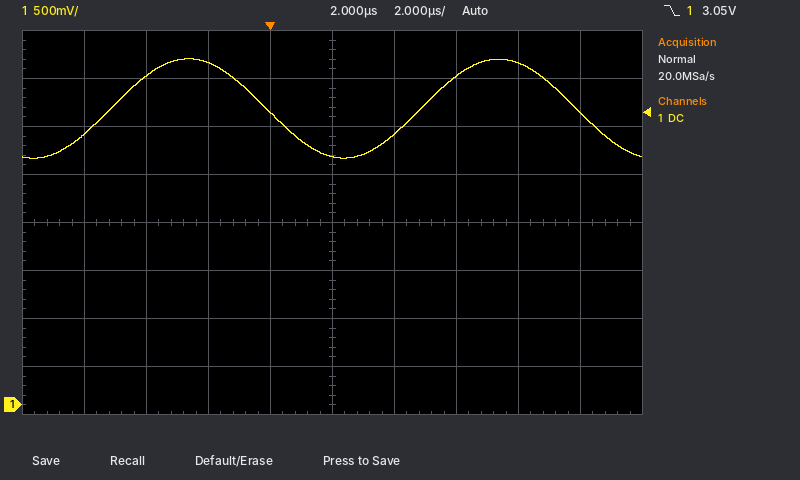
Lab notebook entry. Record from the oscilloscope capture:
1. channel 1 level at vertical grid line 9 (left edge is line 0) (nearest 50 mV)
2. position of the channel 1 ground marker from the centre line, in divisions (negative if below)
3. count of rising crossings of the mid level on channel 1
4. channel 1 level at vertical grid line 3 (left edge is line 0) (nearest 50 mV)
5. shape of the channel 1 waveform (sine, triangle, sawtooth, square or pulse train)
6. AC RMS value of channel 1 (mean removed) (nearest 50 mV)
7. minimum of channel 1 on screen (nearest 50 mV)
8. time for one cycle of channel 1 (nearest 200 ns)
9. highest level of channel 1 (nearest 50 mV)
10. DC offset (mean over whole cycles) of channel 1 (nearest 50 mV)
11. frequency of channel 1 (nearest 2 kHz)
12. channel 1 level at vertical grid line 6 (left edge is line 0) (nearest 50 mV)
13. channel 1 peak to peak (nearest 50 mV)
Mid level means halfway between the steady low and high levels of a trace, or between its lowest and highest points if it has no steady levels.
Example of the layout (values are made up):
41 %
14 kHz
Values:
3.05 V
-3.8 div
2
3.55 V
sine
350 mV
2.55 V
10.0 µs
3.60 V
3.10 V
100 kHz
2.80 V
1.05 V
